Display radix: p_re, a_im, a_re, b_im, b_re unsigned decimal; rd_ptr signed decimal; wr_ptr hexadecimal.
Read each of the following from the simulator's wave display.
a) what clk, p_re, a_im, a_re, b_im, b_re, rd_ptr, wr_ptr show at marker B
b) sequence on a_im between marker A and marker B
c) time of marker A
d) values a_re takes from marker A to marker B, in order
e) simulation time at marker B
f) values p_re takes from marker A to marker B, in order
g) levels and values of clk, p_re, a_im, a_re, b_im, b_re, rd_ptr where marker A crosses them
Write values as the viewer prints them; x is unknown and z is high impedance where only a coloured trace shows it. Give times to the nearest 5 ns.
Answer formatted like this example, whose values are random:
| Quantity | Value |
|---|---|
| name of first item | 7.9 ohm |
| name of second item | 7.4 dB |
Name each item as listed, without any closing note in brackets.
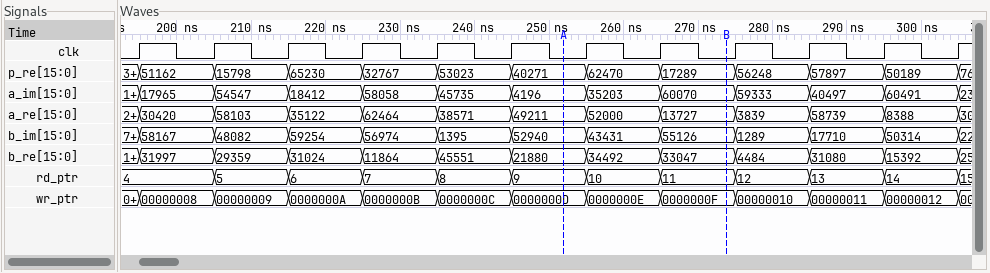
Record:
| Quantity | Value |
|---|---|
| what clk, p_re, a_im, a_re, b_im, b_re, rd_ptr, wr_ptr show at marker B | clk=0, p_re=17289, a_im=60070, a_re=13727, b_im=55126, b_re=33047, rd_ptr=11, wr_ptr=0000000F |
| sequence on a_im between marker A and marker B | 4196, 35203, 60070 |
| time of marker A | 250 ns |
| values a_re takes from marker A to marker B, in order | 49211, 52000, 13727 |
| simulation time at marker B | 275 ns |
| values p_re takes from marker A to marker B, in order | 40271, 62470, 17289 |
| levels and values of clk, p_re, a_im, a_re, b_im, b_re, rd_ptr where marker A crosses them | clk=0, p_re=40271, a_im=4196, a_re=49211, b_im=52940, b_re=21880, rd_ptr=9 |
